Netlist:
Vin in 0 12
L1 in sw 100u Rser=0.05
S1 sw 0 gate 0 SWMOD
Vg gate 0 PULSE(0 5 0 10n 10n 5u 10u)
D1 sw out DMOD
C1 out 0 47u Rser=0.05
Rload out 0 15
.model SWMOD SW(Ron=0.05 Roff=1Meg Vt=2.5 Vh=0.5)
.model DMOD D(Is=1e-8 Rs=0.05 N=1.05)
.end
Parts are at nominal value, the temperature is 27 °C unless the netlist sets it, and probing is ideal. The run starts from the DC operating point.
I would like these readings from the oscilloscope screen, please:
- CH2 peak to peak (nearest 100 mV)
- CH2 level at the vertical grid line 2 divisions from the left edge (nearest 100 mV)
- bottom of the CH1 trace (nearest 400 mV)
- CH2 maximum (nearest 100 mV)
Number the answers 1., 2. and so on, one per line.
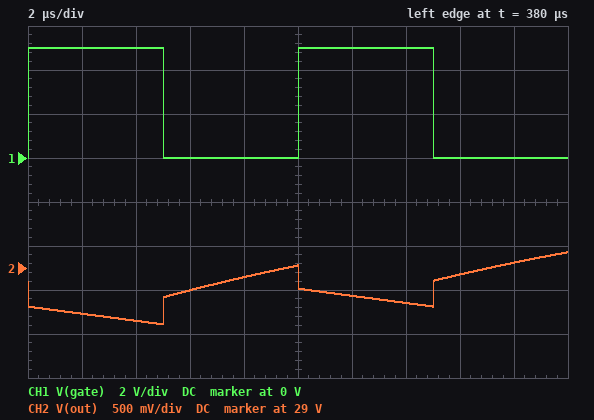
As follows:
1. 800 mV
2. 28.4 V
3. 0 V
4. 29.2 V
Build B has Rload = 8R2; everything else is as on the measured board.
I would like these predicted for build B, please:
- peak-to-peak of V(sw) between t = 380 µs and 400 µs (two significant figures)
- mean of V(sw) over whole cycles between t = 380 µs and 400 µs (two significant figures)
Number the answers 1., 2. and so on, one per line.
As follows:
1. 28 V
2. 14 V
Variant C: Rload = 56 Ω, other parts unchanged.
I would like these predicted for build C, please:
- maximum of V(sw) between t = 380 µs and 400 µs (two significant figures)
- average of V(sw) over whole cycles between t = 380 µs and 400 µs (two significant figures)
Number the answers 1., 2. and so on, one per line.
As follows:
1. 32 V
2. 16 V
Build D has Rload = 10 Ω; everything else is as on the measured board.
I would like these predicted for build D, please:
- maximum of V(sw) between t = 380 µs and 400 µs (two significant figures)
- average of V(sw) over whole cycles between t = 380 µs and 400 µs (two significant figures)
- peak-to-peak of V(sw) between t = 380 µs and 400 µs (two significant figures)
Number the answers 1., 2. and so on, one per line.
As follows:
1. 29 V
2. 14 V
3. 28 V
